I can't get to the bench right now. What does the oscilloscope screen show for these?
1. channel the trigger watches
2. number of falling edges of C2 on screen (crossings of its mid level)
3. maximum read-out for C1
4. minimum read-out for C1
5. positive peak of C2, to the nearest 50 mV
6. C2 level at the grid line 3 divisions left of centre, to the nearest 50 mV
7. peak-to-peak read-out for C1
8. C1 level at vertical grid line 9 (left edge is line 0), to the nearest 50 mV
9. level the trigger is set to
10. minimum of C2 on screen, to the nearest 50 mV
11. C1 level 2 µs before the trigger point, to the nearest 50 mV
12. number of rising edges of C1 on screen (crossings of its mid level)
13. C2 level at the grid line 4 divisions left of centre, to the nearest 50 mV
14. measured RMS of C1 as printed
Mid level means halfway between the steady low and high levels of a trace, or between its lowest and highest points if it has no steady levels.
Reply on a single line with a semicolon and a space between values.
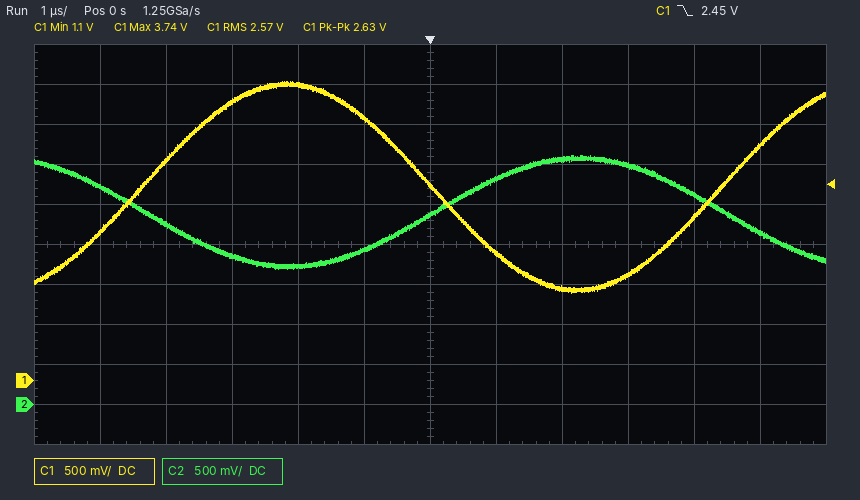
C1; 2; 3.74 V; 1.1 V; 3.10 V; 1.85 V; 2.63 V; 1.30 V; 2.45 V; 1.70 V; 3.70 V; 2; 2.25 V; 2.57 V
